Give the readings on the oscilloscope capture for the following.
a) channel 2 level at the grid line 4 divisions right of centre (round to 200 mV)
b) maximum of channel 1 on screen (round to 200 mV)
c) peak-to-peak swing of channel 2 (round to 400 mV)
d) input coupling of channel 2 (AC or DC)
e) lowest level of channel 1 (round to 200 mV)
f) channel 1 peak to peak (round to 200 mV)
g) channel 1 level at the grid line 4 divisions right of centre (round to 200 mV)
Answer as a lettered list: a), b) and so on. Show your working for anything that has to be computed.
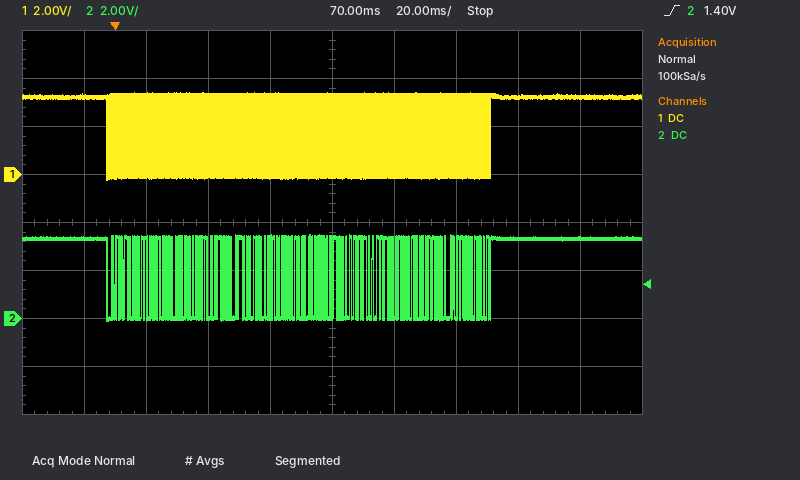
a) 3.4 V
b) 3.4 V
c) 3.6 V
d) DC
e) -200 mV
f) 3.4 V − (-200 mV) = 3.6 V
g) 3.2 V
